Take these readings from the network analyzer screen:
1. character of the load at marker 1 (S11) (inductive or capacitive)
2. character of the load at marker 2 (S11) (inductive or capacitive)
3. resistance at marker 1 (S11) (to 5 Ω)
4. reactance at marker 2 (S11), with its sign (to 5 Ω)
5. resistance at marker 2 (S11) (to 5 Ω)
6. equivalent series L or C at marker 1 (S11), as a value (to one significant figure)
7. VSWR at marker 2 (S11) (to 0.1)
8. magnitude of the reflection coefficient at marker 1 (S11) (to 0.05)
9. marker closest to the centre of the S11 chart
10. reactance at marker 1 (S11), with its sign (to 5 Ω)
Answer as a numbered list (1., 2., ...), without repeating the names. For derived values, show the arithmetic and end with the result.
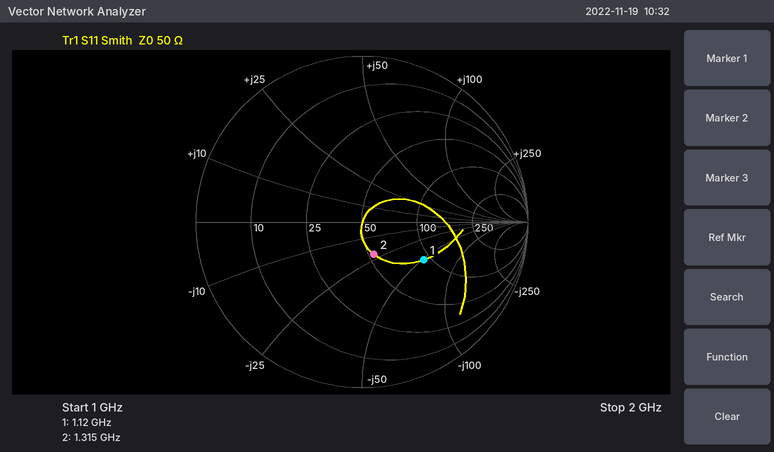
1. capacitive
2. capacitive
3. 90 Ω
4. -20 Ω
5. 55 Ω
6. C = 1/(2π × 1.12 GHz × 50 Ω) ≈ 3 pF
7. 1.5
8. 0.45
9. marker 2
10. -50 Ω
